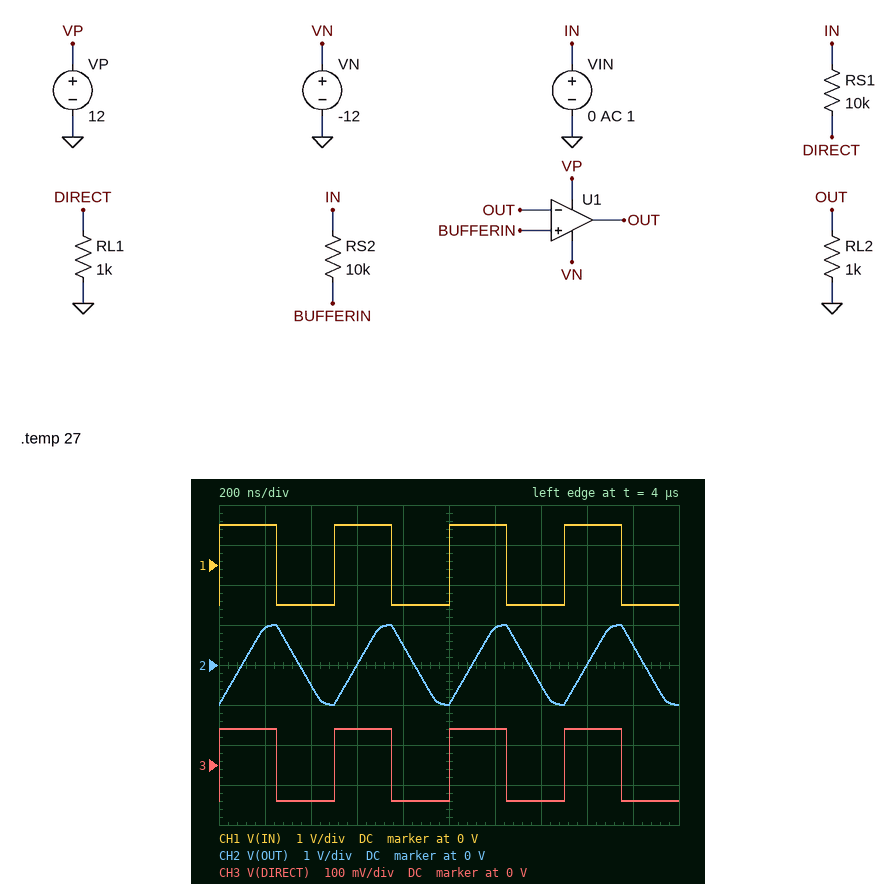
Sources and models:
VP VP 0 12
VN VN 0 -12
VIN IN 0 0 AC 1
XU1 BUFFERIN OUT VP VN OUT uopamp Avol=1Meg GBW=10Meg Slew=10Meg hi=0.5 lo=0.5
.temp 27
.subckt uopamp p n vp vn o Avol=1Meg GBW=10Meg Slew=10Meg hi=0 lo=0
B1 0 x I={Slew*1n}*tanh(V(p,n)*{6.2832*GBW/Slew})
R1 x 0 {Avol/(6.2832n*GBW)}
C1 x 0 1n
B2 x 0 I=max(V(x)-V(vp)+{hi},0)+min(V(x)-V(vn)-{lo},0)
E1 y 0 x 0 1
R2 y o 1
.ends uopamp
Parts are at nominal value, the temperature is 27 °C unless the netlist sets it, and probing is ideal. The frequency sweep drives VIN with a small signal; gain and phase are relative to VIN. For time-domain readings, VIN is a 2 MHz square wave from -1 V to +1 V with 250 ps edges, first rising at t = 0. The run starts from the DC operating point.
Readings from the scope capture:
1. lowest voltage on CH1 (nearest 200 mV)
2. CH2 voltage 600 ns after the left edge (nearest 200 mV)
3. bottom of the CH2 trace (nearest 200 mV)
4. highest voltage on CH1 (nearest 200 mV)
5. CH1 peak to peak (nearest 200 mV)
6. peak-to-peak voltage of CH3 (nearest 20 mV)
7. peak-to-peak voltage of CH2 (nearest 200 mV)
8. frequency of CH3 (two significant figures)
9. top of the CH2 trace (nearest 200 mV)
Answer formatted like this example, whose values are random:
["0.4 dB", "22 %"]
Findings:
["-1.0 V", "0 V", "-1.0 V", "1.0 V", "2.0 V", "180 mV", "2.0 V", "2.0 MHz", "1.0 V"]
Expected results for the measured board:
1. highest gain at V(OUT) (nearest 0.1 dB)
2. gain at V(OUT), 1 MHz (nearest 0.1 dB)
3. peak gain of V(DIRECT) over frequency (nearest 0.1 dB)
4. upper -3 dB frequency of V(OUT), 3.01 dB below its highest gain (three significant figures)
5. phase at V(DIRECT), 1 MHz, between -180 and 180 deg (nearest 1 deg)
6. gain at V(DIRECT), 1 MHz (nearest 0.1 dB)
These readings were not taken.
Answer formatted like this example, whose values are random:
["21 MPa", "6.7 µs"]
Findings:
["0 dB", "0 dB", "-20.8 dB", "9.99 MHz", "0 deg", "-20.8 dB"]
